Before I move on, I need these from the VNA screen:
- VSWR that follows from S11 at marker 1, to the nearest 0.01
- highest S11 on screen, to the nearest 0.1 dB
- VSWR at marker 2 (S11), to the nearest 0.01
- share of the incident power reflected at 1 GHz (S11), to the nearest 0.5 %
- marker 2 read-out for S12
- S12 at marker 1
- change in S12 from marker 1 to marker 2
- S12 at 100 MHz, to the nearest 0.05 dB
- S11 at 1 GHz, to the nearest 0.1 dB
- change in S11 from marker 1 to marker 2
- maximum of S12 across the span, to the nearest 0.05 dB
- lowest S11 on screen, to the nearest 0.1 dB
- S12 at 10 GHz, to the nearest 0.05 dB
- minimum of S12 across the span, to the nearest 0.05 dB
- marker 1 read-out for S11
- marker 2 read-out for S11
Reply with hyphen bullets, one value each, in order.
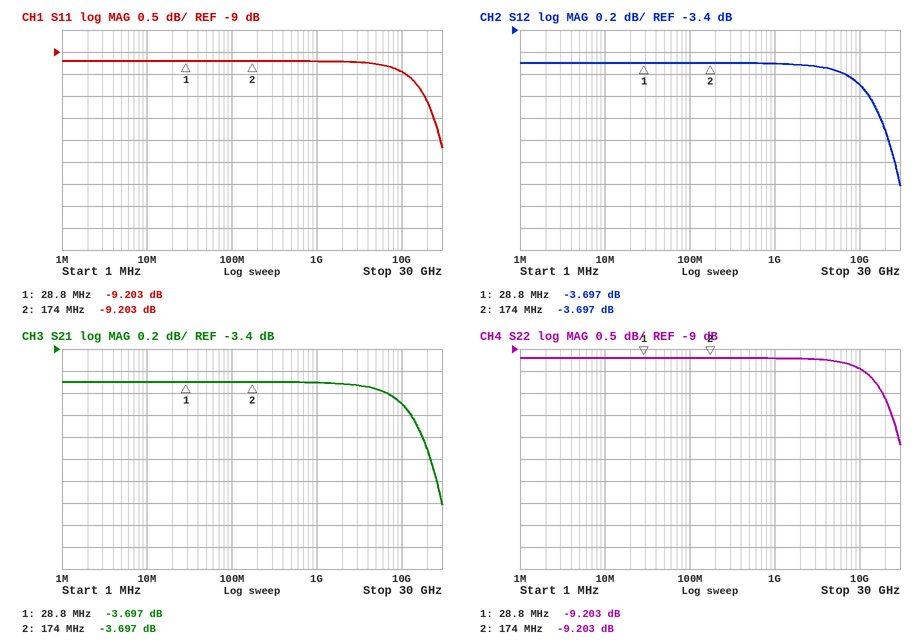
- 2.06
- -9.2 dB
- 2.06
- 12.0 %
- -3.697 dB
- -3.697 dB
- 0.000 dB
- -3.70 dB
- -9.2 dB
- 0.000 dB
- -3.70 dB
- -11.2 dB
- -3.90 dB
- -4.80 dB
- -9.203 dB
- -9.203 dB
